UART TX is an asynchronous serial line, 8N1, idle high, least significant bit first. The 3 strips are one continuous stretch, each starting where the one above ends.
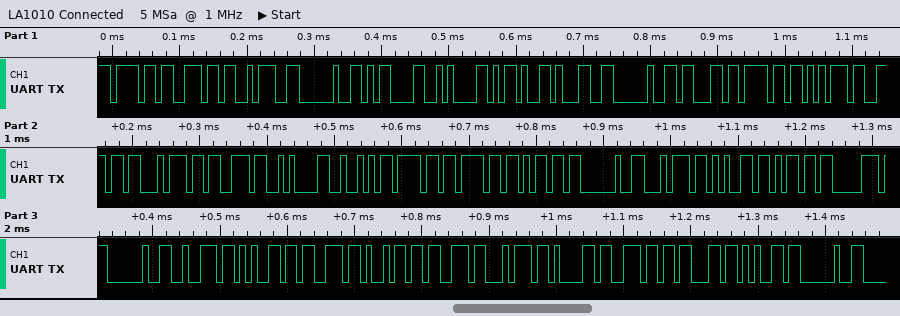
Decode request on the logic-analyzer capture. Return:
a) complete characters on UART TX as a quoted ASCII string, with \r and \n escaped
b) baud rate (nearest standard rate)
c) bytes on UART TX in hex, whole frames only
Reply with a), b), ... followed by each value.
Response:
a) "on: \r\n-1 counts\nRoom temp resistance "
b) 115200 baud
c) 6F 6E 3A 20 0D 0A 2D 31 20 63 6F 75 6E 74 73 0A 52 6F 6F 6D 20 74 65 6D 70 20 72 65 73 69 73 74 61 6E 63 65 20
